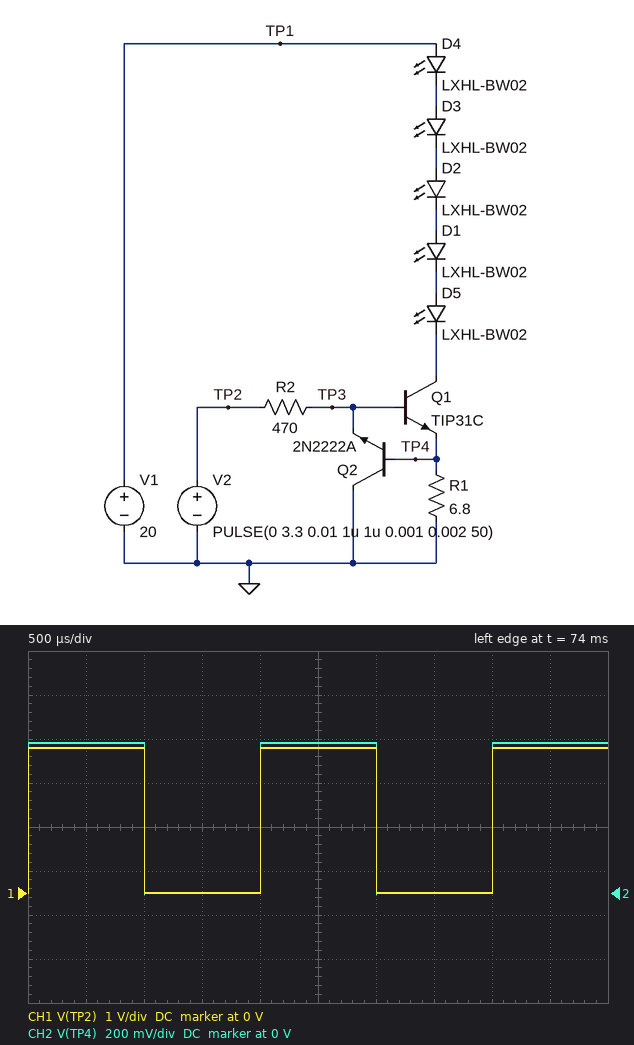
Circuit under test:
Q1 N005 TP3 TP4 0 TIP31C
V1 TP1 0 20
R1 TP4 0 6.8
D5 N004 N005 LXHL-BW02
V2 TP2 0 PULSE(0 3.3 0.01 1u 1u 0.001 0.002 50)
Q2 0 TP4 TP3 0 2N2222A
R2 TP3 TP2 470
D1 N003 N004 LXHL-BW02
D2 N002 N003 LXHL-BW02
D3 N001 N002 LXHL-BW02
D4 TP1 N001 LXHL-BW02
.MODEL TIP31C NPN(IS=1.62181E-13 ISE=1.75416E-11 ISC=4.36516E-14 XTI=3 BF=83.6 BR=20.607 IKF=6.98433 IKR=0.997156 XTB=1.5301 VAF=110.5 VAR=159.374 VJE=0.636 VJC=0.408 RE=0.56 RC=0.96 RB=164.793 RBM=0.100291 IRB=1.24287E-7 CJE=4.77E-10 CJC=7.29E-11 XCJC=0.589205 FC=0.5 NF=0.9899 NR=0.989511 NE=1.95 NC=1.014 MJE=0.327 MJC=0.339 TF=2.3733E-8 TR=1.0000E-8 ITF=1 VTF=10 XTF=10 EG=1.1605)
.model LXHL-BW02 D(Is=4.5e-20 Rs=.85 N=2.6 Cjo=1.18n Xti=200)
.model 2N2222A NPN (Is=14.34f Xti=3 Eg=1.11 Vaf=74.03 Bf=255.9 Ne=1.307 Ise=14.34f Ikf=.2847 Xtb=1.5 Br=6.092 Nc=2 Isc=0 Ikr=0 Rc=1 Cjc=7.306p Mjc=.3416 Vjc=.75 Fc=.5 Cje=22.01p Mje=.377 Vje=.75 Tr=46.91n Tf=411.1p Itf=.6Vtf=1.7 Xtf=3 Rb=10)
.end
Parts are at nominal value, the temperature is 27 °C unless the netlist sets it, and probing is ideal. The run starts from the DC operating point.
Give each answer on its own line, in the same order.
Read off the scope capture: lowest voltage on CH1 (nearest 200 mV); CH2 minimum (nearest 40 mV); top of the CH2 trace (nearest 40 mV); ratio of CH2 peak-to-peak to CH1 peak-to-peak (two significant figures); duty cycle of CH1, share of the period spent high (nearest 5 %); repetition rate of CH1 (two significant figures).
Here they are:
0 V
0 V
680 mV
0.21
50 %
500 Hz
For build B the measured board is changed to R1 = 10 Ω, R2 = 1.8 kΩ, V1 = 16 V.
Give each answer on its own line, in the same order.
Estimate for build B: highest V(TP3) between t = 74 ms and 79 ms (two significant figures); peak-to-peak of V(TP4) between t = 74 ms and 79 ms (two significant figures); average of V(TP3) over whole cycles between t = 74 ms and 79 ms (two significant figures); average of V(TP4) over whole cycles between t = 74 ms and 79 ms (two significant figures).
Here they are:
1.3 V
620 mV
670 mV
310 mV
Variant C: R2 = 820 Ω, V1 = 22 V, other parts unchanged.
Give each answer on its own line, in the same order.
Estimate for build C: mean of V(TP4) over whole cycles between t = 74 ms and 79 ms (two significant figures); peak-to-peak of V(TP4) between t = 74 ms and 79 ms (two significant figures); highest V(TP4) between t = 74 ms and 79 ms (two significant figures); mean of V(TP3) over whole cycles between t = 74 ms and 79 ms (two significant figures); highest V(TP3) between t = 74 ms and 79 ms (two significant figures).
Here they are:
330 mV
660 mV
650 mV
700 mV
1.4 V
